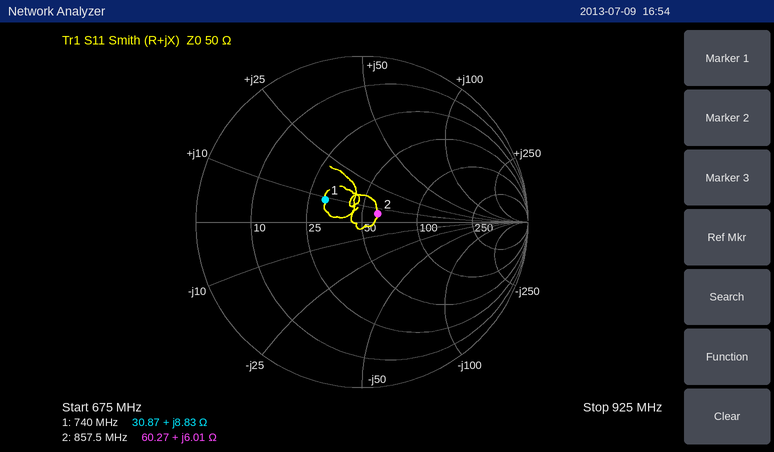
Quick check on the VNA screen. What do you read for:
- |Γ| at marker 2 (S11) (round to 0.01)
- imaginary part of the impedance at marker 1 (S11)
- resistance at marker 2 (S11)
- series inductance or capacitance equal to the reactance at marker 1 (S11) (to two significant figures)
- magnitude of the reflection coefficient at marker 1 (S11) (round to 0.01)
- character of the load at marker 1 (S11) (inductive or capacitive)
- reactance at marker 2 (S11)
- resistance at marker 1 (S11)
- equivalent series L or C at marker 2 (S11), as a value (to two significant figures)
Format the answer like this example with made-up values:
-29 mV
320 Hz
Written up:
0.11
+8.83 Ω
60.27 Ω
1.9 nH
0.26
inductive
+6.01 Ω
30.87 Ω
1.1 nH
